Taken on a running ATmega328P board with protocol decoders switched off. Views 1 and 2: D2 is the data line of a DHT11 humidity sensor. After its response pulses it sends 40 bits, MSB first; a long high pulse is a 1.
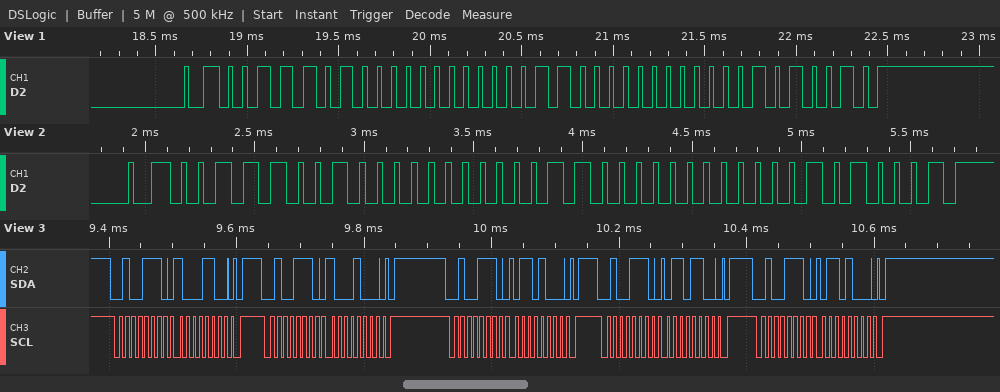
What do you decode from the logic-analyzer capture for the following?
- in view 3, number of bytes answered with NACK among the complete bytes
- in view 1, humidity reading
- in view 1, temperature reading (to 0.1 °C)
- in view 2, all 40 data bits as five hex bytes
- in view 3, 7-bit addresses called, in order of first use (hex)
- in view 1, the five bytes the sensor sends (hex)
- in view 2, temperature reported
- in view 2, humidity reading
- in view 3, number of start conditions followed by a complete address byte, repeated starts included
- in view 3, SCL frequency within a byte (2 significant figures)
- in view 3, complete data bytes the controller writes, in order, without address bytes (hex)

0
58 %
24.0 °C
39 00 18 00 51
0x27
3A 00 18 00 52
24.0 °C
57 %
5
100 kHz
8C 88 68 6C 68
